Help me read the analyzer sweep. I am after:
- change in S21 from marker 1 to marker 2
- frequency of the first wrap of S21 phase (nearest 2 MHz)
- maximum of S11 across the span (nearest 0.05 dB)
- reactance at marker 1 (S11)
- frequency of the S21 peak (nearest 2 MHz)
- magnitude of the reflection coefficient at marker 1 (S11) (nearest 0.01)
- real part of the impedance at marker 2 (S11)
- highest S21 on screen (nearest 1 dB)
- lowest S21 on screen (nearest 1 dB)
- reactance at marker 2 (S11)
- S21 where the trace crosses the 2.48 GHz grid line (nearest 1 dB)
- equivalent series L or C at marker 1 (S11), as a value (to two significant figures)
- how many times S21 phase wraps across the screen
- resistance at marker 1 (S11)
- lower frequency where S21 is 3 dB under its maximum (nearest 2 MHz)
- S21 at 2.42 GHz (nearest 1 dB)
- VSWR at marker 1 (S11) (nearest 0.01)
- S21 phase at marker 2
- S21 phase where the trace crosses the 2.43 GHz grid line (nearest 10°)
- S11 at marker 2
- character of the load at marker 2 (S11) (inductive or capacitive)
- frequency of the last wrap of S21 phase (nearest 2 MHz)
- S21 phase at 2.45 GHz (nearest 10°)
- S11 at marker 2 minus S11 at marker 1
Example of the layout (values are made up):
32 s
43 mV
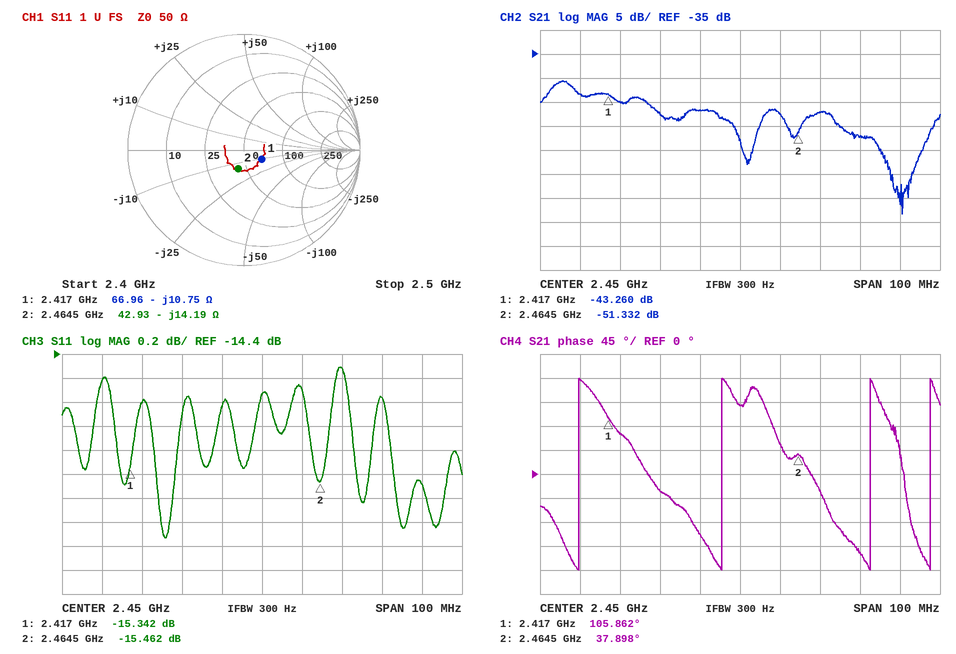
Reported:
-8.072 dB
2.410 GHz
-14.50 dB
-10.75 Ω
2.406 GHz
0.17
42.93 Ω
-41 dB
-68 dB
-14.19 Ω
-52 dB
6.1 pF
4
66.96 Ω
2.402 GHz
-45 dB
1.41
37.898°
-30°
-15.462 dB
capacitive
2.498 GHz
130°
-0.120 dB
